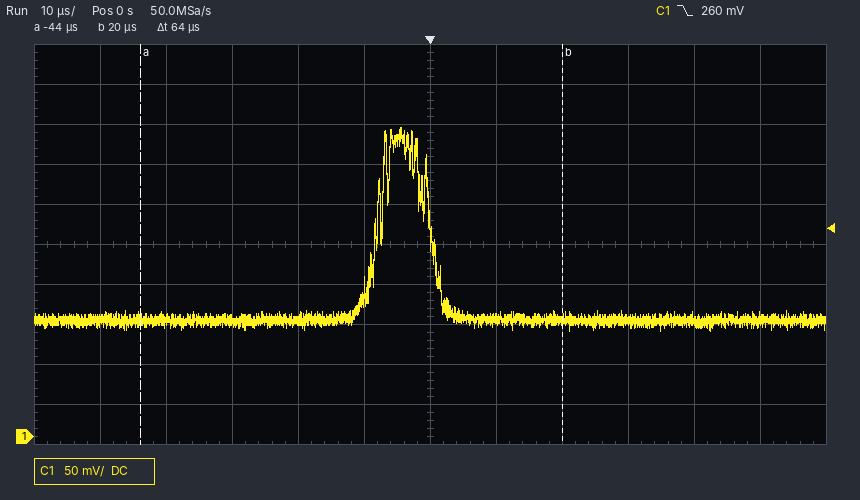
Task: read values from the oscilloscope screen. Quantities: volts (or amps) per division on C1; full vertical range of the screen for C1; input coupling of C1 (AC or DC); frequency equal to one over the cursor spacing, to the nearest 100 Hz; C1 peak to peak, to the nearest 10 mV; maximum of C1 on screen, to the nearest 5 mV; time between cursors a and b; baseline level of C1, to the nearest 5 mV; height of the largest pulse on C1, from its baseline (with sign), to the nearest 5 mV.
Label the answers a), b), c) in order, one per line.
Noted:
a) 50 mV
b) 500 mV
c) DC
d) 15.6 kHz
e) 250 mV
f) 385 mV
g) 64 µs
h) 145 mV
i) +240 mV
